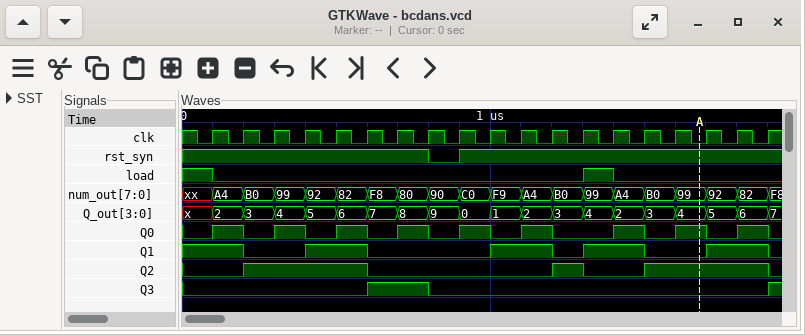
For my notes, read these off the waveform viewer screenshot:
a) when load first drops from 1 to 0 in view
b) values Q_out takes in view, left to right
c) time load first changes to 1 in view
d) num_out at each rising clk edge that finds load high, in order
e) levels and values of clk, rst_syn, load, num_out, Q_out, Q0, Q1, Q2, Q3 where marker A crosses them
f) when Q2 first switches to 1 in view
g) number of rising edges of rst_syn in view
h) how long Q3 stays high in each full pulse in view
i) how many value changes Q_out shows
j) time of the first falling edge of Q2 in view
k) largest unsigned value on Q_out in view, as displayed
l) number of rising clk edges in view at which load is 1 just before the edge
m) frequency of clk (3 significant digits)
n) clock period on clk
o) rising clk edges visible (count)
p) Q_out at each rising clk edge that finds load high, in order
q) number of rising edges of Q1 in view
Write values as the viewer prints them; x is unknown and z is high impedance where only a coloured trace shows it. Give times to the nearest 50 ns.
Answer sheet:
100 ns
x, 2, 3, 4, 5, 6, 7, 8, 9, 0, 1, 2, 3, 4, 2, 3, 4, 5, 6, 7
1300 ns
xx, 99
clk=0, rst_syn=1, load=0, num_out=99, Q_out=4, Q0=1, Q1=0, Q2=1, Q3=0
200 ns
1
200 ns
19
600 ns
9
2
10.0 MHz
100 ns
19
x, 4
4
